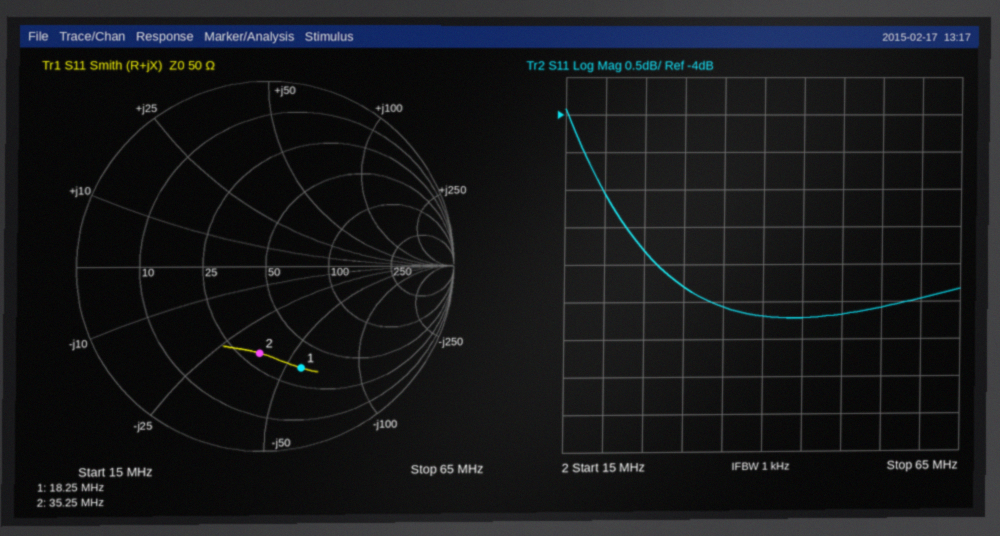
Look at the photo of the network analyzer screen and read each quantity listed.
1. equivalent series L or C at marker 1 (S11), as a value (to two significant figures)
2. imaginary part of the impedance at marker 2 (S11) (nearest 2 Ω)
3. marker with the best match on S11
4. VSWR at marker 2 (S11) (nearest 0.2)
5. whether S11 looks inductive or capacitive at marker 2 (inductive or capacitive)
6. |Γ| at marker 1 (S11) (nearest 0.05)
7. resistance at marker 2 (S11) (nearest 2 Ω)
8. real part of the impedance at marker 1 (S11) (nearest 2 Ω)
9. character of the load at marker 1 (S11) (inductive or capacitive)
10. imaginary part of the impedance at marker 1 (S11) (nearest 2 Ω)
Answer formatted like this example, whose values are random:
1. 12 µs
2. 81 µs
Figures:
1. 150 pF
2. -36 Ω
3. marker 2
4. 2.8
5. capacitive
6. 0.60
7. 30 Ω
8. 34 Ω
9. capacitive
10. -58 Ω
